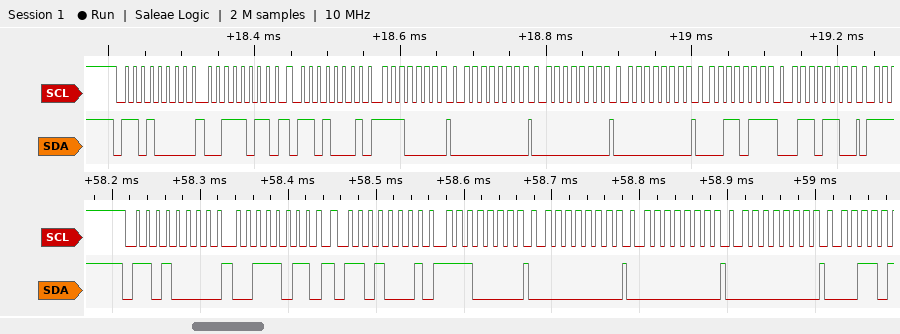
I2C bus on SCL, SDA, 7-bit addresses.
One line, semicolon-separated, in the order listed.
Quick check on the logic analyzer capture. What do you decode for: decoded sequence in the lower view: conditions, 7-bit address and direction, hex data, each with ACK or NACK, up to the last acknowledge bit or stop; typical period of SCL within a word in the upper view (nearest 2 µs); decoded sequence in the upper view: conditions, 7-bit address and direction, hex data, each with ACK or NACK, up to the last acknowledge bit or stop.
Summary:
start, address 68 write ACK, 3B ACK, repeated start, address 68 read ACK, E0 ACK, 00 ACK, 00 ACK, 00 ACK; 12 µs; start, address 68 write ACK, 3B ACK, repeated start, address 68 read ACK, E0 ACK, 00 ACK, 00 ACK, 00 ACK, 37 ACK, 6C ACK
